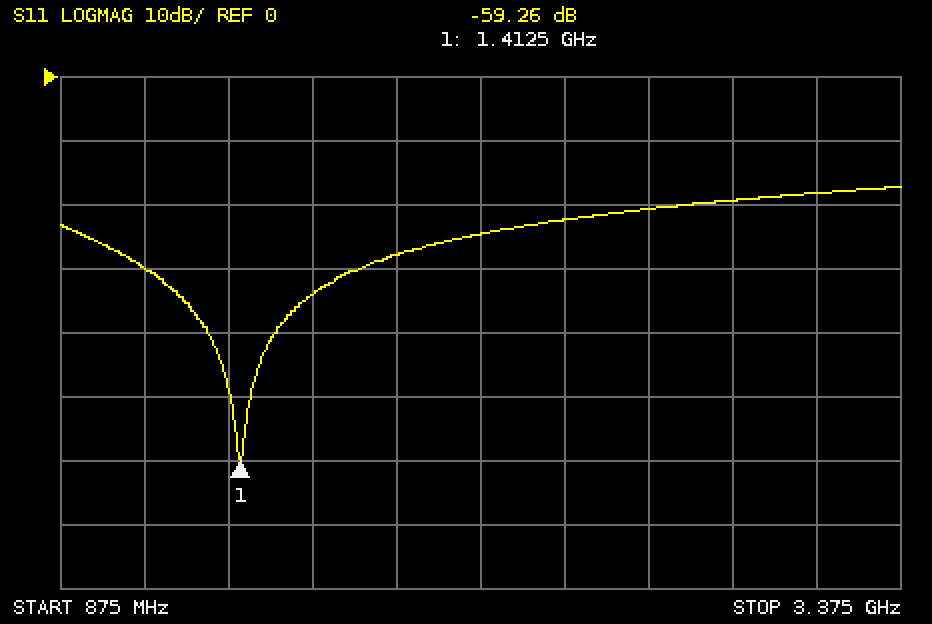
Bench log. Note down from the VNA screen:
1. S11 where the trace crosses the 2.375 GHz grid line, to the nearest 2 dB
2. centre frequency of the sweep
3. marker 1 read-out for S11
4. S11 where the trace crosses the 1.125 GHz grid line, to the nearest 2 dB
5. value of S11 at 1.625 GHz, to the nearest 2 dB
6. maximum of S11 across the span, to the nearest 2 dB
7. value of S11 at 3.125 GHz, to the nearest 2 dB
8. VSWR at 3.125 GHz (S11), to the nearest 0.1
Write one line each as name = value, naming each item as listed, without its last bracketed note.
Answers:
S11 where the trace crosses the 2.375 GHz grid line, to the nearest 2 dB = -22 dB
centre frequency of the sweep = 2.125 GHz
marker 1 read-out for S11 = -59.26 dB
S11 where the trace crosses the 1.125 GHz grid line, to the nearest 2 dB = -30 dB
value of S11 at 1.625 GHz, to the nearest 2 dB = -34 dB
maximum of S11 across the span, to the nearest 2 dB = -18 dB
value of S11 at 3.125 GHz, to the nearest 2 dB = -18 dB
VSWR at 3.125 GHz (S11), to the nearest 0.1 = 1.3
